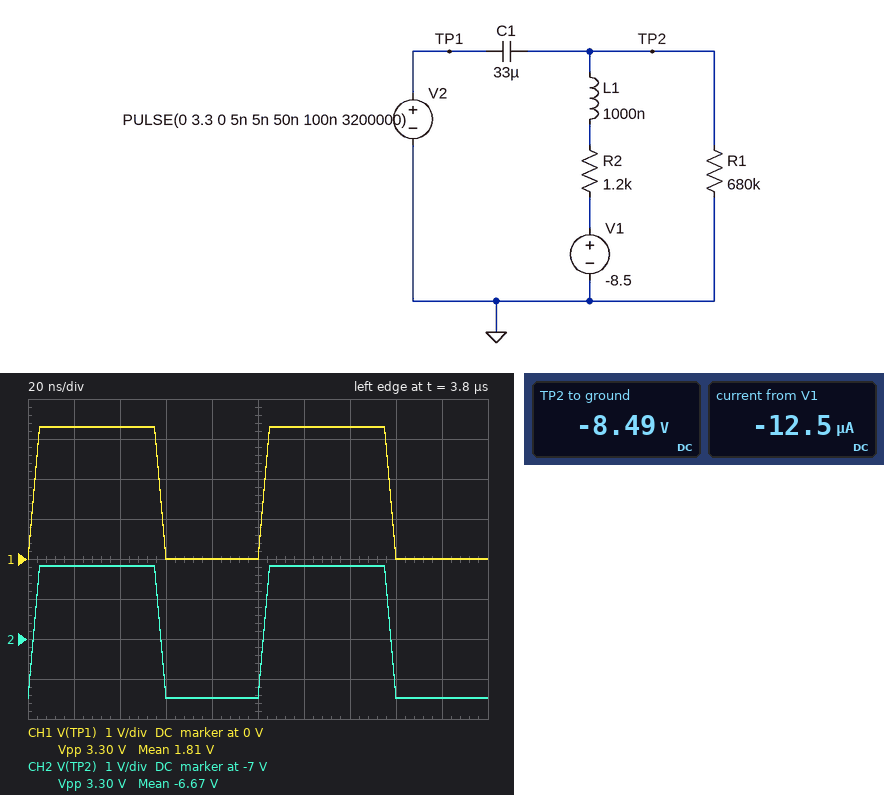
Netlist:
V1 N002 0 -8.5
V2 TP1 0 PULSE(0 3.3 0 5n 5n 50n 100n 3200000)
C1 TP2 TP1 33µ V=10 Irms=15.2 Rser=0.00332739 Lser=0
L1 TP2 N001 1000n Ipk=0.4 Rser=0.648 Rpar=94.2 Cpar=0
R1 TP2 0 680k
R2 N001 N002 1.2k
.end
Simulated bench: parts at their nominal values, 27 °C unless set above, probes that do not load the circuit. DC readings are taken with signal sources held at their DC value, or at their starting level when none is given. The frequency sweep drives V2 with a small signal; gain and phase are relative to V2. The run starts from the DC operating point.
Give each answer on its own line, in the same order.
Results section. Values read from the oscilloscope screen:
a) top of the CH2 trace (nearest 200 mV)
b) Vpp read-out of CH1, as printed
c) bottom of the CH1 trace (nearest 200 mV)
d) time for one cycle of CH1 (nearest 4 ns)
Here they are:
-5.2 V
3.30 V
0 V
100 ns
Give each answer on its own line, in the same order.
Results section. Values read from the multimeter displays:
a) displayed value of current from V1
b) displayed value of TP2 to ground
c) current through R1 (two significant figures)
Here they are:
-12.5 µA
-8.49 V
12 µA
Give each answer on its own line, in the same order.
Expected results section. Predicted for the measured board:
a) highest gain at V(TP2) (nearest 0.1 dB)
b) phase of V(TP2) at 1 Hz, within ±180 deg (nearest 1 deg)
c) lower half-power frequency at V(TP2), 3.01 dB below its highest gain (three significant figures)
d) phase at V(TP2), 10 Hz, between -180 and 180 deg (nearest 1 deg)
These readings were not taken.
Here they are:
0 dB
76 deg
4.02 Hz
22 deg
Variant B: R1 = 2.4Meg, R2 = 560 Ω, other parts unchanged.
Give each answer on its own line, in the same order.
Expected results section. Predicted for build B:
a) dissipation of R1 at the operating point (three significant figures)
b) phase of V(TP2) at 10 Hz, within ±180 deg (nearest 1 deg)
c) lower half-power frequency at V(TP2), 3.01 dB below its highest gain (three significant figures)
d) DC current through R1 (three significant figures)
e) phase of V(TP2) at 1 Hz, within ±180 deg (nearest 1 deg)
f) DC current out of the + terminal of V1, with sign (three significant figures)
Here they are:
30.1 µW
41 deg
8.60 Hz
3.54 µA
83 deg
-3.54 µA
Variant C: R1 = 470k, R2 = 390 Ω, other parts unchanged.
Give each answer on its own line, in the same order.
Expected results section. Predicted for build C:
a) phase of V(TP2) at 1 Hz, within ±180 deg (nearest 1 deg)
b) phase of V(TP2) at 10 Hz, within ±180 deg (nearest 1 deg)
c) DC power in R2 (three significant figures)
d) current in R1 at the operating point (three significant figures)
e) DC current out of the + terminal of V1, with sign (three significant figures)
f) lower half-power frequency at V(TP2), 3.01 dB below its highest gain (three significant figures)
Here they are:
85 deg
51 deg
127 nW
18.1 µA
-18.1 µA
12.4 Hz
